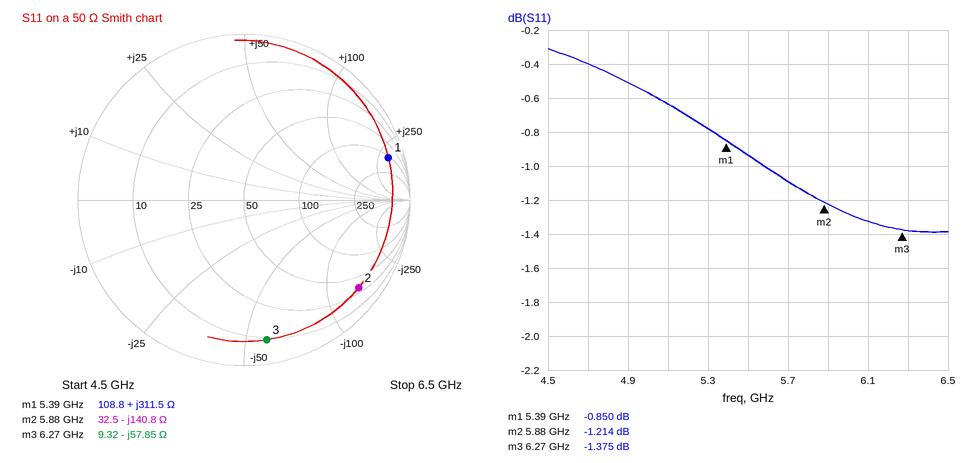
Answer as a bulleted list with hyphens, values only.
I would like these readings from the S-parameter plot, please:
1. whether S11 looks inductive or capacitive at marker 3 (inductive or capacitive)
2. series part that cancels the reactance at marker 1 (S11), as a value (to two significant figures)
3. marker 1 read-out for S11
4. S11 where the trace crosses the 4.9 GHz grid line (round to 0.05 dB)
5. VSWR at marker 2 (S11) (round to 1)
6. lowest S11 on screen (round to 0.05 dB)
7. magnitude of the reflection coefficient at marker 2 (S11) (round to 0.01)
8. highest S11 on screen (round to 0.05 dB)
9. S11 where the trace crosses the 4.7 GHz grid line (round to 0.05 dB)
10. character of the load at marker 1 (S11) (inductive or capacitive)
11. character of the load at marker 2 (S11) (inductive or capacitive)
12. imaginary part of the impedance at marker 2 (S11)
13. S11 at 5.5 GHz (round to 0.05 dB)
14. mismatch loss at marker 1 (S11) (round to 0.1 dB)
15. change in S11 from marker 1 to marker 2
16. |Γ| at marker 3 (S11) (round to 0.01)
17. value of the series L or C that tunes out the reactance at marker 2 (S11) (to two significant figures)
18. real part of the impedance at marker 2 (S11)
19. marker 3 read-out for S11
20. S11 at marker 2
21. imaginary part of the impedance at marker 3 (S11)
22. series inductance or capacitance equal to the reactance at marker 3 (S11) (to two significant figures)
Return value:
- capacitive
- 95 fF
- -0.850 dB
- -0.50 dB
- 14
- -1.40 dB
- 0.87
- -0.30 dB
- -0.40 dB
- inductive
- capacitive
- -140.8 Ω
- -0.95 dB
- 7.5 dB
- -0.364 dB
- 0.85
- 3.8 nH
- 32.5 Ω
- -1.375 dB
- -1.214 dB
- -57.85 Ω
- 440 fF
